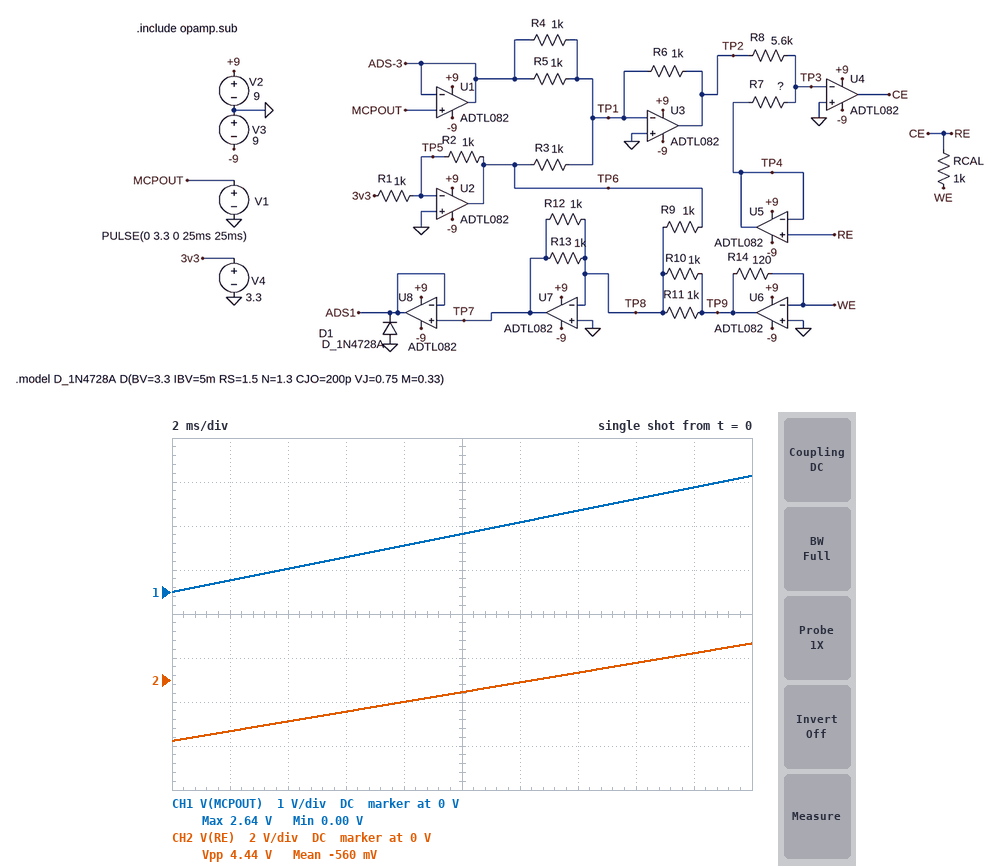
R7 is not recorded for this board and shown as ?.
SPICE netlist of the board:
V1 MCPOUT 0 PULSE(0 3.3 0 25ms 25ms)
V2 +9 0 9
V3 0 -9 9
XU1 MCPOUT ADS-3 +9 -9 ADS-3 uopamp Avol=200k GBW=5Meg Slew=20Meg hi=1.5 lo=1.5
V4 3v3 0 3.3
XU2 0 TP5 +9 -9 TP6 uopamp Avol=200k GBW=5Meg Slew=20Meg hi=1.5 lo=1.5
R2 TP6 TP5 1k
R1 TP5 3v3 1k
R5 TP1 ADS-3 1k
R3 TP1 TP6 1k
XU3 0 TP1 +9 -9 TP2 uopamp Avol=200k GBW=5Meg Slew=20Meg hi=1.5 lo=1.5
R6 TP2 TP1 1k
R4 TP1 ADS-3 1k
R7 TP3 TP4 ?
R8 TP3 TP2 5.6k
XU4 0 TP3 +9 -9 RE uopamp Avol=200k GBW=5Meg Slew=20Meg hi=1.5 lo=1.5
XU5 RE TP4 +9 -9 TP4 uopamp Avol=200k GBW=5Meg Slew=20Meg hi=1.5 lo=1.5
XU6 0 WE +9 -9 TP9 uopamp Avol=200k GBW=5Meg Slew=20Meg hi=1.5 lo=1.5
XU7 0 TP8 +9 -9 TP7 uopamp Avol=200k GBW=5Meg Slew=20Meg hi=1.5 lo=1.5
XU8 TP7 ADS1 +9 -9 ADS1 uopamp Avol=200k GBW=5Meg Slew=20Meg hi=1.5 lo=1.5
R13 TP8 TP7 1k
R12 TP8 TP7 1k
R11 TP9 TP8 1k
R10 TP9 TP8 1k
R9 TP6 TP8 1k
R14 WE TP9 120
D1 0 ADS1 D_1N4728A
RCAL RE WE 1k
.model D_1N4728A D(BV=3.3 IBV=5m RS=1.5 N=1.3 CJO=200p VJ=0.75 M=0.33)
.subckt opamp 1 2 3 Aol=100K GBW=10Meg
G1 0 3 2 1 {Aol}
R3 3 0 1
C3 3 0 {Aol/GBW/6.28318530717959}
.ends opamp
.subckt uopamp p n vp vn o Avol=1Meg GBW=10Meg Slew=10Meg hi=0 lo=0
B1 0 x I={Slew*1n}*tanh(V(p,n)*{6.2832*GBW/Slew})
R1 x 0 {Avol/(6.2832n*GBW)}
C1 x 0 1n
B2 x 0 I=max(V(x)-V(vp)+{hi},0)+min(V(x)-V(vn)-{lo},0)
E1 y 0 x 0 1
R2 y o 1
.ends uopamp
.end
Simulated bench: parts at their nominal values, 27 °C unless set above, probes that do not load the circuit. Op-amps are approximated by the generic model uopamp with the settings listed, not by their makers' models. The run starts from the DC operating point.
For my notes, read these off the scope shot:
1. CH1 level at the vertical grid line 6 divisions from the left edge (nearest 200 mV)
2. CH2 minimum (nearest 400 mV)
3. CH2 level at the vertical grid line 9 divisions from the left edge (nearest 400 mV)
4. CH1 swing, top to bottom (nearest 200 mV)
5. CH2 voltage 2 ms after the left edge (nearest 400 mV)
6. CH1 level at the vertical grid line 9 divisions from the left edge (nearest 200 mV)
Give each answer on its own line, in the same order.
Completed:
1.6 V
-2.8 V
1.2 V
2.6 V
-2.4 V
2.4 V
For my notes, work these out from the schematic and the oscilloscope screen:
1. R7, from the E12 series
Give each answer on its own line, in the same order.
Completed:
4.7 kΩ
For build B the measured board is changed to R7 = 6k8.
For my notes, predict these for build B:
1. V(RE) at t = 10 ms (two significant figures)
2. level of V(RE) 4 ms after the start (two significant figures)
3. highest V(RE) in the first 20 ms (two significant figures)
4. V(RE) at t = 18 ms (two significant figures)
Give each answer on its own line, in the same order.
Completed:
-800 mV
-2.7 V
2.4 V
1.8 V
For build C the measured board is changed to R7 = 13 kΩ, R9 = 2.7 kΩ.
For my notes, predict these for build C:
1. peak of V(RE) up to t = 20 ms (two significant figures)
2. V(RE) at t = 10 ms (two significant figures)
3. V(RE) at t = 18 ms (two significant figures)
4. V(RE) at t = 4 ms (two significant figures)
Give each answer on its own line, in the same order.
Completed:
4.6 V
-1.5 V
3.4 V
-5.2 V
